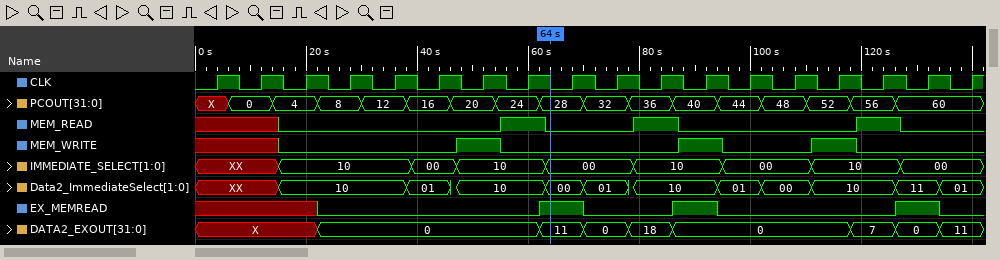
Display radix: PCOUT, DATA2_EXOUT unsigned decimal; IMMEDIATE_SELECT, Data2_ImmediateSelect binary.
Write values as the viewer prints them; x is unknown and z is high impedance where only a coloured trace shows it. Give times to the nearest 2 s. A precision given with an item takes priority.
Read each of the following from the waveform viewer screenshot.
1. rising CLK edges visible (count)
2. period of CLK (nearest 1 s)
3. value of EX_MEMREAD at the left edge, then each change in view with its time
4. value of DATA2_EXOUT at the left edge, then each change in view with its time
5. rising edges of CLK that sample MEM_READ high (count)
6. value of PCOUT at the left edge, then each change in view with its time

18
8 s
x, 0 at 22 s, 1 at 62 s, 0 at 70 s, 1 at 86 s, 0 at 94 s, 1 at 126 s, 0 at 134 s
X, 0 at 22 s, 11 at 62 s, 0 at 70 s, 18 at 78 s, 0 at 86 s, 7 at 118 s, 0 at 126 s, 11 at 134 s
3
X, 0 at 6 s, 4 at 14 s, 8 at 22 s, 12 at 30 s, 16 at 38 s, 20 at 46 s, 24 at 54 s, 28 at 62 s, 32 at 70 s, 36 at 78 s, 40 at 86 s, 44 at 94 s, 48 at 102 s, 52 at 110 s, 56 at 118 s, 60 at 126 s
